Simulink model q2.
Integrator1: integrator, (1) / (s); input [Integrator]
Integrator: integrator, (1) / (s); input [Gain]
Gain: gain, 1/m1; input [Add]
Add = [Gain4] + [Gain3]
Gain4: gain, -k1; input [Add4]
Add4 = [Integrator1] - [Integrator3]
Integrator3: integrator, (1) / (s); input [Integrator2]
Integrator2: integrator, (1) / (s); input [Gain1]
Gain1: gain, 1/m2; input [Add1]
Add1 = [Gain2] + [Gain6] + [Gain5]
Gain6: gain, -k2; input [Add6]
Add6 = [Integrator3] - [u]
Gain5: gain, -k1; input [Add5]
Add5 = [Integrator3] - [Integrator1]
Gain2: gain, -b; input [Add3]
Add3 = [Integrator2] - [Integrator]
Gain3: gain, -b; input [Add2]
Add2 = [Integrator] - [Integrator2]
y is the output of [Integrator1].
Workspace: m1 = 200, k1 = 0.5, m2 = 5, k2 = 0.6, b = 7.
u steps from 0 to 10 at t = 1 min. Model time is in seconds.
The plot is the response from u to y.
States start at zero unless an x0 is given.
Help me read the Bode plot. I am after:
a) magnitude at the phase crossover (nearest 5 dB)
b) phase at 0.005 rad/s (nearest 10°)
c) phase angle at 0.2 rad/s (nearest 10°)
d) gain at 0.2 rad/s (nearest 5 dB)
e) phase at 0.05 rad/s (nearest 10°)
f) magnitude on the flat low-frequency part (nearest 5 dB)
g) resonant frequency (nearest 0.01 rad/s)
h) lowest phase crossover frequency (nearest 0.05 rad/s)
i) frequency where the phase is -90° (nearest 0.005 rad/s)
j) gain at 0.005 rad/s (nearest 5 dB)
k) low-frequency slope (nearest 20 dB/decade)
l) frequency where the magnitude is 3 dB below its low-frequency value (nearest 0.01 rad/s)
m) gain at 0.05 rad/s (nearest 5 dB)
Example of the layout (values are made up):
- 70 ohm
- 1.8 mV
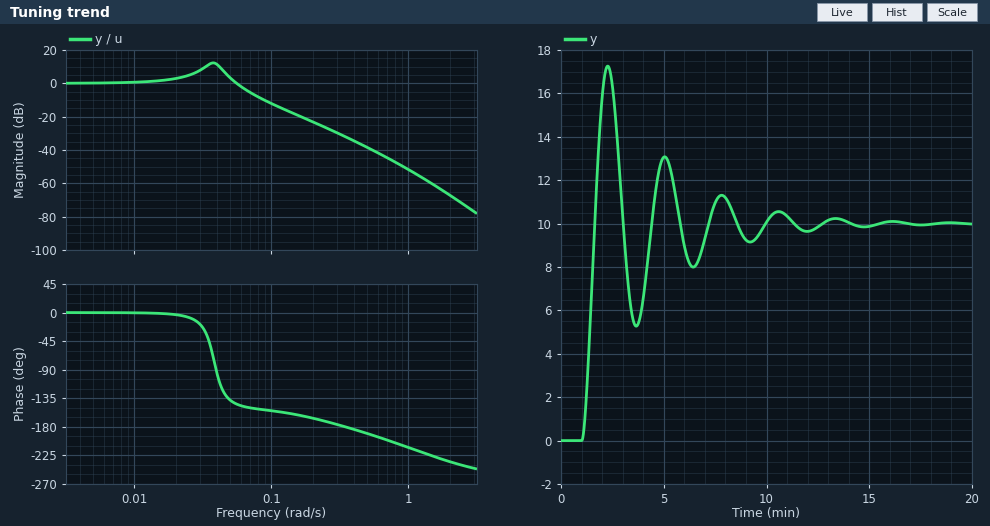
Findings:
- -30 dB
- 0°
- -170°
- -25 dB
- -140°
- 0 dB
- 0.04 rad/s
- 0.35 rad/s
- 0.040 rad/s
- 0 dB
- 0 dB/decade
- 0.06 rad/s
- 5 dB
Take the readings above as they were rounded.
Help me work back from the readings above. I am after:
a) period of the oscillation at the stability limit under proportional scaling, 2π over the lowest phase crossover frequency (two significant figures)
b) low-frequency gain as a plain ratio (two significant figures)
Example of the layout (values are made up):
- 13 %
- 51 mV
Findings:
- 18 s
- 1.0
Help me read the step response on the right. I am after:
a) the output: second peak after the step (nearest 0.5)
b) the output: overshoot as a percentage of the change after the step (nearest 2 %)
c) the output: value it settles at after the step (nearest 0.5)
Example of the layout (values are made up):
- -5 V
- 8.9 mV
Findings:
- 13.0
- 72 %
- 10.0
